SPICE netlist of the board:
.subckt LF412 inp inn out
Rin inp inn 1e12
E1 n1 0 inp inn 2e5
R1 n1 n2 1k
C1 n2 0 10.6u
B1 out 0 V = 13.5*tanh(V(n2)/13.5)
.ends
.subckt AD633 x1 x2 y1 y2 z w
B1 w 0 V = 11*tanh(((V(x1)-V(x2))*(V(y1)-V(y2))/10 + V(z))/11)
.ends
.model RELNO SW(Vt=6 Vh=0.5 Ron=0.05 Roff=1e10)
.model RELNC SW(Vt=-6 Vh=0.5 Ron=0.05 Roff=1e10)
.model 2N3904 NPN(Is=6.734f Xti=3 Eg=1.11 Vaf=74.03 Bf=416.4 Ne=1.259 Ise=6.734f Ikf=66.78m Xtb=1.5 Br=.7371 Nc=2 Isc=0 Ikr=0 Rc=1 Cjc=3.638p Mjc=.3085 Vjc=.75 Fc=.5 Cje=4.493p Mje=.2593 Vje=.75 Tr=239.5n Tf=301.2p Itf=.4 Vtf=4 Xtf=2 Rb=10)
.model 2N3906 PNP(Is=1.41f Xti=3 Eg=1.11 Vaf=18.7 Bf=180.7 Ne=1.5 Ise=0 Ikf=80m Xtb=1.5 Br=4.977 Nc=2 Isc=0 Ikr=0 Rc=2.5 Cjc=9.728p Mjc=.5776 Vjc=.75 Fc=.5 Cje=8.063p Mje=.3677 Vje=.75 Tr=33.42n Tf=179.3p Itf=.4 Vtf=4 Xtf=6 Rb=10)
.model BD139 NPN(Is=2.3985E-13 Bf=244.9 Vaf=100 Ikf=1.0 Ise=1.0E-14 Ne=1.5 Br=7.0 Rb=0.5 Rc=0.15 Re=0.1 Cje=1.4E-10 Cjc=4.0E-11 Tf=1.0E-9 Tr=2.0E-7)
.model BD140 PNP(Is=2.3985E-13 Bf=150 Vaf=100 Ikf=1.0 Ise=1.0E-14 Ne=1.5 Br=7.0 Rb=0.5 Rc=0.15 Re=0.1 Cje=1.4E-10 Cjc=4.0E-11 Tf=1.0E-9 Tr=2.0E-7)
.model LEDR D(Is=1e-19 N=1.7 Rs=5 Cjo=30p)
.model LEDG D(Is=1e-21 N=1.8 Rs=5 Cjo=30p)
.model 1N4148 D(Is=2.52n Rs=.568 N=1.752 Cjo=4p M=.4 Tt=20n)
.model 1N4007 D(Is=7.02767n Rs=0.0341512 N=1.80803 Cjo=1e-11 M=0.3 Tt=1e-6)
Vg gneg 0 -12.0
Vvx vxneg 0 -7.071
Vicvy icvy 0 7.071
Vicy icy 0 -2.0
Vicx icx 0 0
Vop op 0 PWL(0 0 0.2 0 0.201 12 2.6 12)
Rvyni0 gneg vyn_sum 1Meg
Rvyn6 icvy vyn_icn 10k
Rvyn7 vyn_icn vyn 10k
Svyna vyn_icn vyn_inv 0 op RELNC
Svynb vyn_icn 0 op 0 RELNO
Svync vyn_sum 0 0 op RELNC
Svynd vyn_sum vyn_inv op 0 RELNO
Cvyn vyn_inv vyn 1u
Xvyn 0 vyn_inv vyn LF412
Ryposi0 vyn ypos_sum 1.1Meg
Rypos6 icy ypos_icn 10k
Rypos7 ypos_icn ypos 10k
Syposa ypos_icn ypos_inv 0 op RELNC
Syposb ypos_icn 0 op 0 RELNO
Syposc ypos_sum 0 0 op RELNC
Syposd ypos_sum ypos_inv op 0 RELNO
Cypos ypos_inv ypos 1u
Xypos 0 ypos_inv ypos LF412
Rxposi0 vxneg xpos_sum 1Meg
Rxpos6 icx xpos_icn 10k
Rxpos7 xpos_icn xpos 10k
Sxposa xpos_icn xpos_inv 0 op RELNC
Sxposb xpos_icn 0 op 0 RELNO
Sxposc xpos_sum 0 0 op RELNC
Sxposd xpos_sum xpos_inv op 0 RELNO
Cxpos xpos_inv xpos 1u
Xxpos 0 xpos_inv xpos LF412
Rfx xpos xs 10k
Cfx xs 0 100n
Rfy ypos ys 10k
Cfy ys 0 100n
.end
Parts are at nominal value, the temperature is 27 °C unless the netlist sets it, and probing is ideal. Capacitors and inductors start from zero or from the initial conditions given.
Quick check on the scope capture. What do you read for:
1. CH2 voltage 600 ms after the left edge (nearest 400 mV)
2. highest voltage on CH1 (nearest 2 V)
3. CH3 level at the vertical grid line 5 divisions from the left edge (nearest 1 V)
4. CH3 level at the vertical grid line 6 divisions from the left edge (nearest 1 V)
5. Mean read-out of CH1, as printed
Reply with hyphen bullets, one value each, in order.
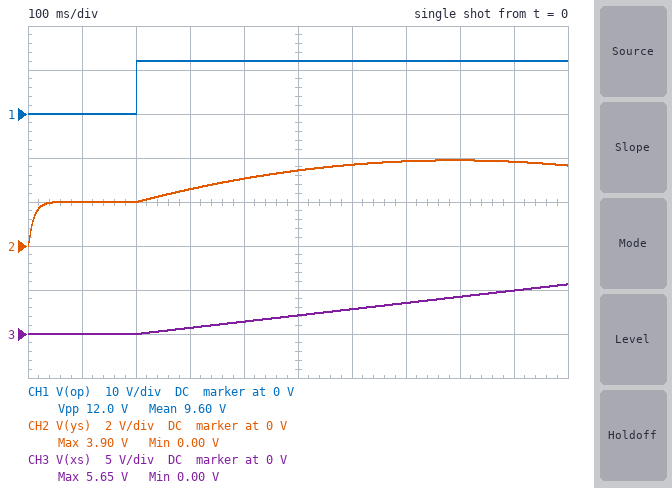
- 3.6 V
- 12 V
- 2 V
- 3 V
- 9.60 V
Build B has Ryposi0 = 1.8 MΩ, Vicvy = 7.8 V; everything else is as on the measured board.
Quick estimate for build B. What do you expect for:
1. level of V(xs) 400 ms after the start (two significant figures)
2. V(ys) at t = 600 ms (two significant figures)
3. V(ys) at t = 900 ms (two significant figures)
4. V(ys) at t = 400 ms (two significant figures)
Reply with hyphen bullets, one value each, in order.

- 1.4 V
- 3.2 V
- 3.4 V
- 2.7 V
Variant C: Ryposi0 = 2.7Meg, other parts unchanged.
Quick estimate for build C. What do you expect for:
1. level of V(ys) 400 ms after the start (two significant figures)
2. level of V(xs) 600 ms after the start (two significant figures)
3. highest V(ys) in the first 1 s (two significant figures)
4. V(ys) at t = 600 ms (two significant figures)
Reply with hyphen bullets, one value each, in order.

- 2.4 V
- 2.8 V
- 2.8 V
- 2.7 V
